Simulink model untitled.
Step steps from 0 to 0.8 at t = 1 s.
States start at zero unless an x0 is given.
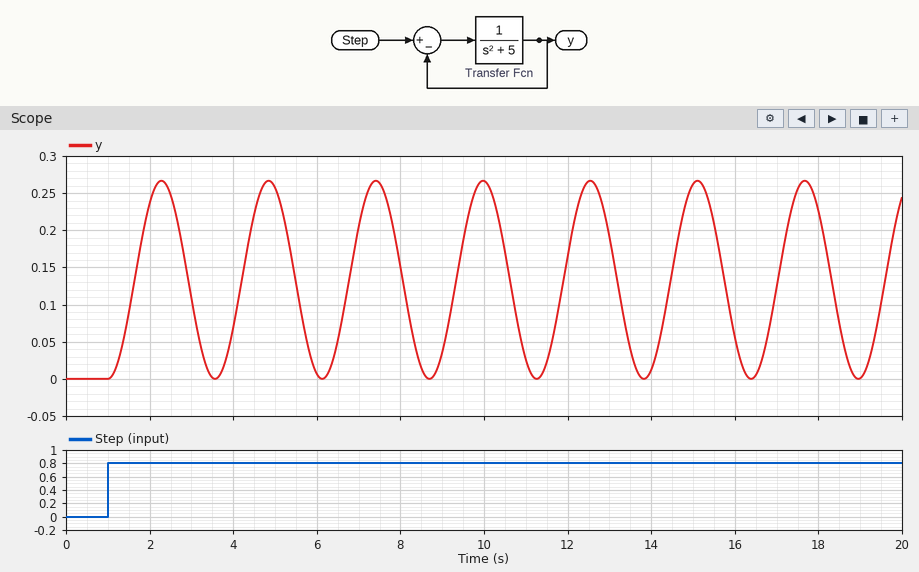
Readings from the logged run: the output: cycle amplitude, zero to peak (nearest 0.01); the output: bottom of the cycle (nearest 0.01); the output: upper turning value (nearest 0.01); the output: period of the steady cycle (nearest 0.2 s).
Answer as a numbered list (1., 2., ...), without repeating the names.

1. 0.13
2. 0.00
3. 0.27
4. 2.6 s
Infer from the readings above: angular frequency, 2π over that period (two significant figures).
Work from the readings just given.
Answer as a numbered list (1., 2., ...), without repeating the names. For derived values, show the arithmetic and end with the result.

1. 2π / 2.6 = 2.4 rad/s
